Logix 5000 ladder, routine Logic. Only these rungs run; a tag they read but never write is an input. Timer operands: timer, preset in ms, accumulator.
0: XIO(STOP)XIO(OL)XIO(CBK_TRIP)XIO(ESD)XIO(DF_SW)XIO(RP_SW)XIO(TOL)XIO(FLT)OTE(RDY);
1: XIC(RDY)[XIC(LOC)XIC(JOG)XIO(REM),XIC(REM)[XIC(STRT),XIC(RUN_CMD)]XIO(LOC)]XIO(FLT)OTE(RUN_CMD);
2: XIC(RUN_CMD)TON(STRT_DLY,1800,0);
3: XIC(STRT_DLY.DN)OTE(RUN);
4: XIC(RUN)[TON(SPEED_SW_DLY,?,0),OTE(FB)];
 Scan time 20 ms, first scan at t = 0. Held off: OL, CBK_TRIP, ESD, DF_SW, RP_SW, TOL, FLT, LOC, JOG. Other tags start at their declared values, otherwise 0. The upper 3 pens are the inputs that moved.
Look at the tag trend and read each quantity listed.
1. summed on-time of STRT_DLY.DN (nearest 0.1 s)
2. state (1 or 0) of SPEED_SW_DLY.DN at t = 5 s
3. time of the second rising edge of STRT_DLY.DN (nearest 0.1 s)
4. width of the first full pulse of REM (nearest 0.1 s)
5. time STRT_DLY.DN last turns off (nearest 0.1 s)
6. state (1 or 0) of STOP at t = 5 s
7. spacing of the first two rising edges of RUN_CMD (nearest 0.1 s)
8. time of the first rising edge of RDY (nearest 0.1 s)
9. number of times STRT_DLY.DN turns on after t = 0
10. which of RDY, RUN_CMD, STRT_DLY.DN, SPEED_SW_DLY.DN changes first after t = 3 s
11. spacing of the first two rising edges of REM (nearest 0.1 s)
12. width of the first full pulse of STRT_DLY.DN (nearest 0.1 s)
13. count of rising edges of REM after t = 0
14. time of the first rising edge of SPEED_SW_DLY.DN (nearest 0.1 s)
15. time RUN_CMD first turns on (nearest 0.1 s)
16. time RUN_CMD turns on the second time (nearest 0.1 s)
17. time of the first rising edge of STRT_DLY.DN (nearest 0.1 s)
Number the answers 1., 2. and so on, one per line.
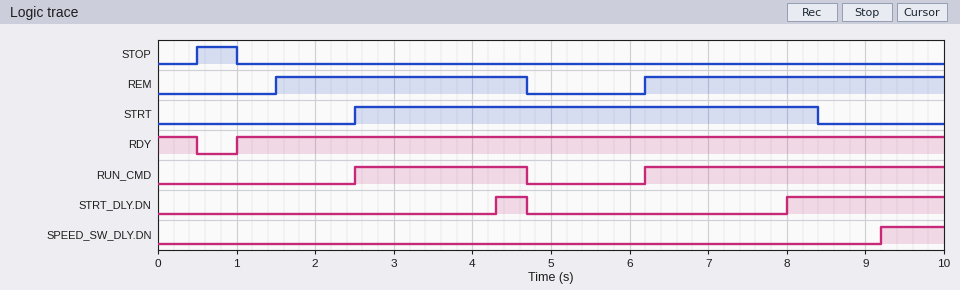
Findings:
1. 2.4 s
2. 0
3. 8.0 s
4. 3.2 s
5. 4.7 s
6. 0
7. 3.7 s
8. 1.0 s
9. 2
10. STRT_DLY.DN
11. 4.7 s
12. 0.4 s
13. 2
14. 9.2 s
15. 2.5 s
16. 6.2 s
17. 4.3 s
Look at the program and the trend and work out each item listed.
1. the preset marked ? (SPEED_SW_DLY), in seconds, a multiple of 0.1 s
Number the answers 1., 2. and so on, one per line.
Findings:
1. 1.2 s
